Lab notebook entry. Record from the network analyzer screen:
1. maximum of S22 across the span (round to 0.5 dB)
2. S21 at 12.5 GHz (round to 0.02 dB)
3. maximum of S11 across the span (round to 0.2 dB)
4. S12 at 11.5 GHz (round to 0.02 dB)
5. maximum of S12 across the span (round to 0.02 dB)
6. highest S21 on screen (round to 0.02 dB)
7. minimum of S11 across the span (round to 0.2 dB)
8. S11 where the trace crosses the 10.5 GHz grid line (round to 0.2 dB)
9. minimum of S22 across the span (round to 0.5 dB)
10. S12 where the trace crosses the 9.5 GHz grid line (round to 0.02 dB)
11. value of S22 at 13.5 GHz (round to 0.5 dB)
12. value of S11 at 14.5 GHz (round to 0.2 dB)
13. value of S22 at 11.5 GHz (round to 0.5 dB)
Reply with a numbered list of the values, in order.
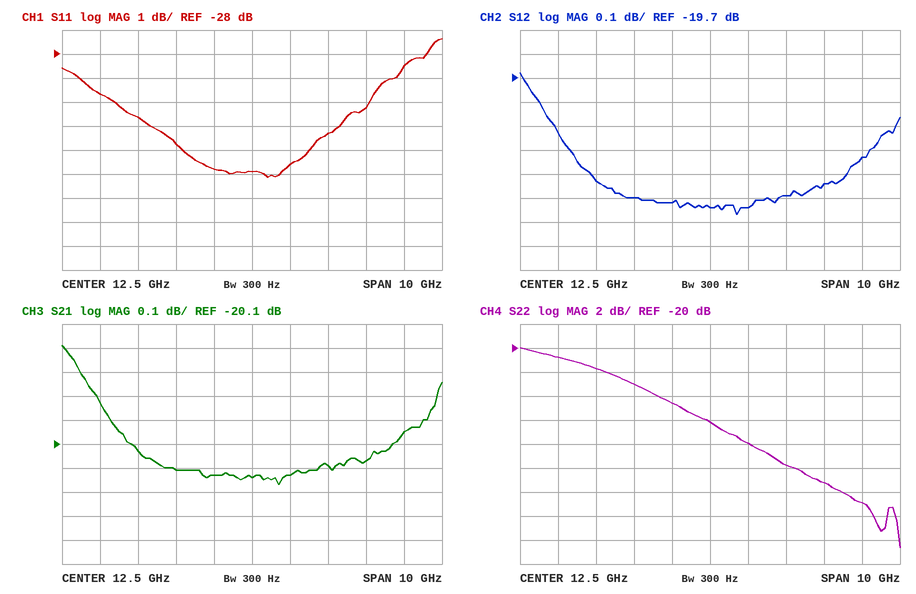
1. -20.0 dB
2. -20.24 dB
3. -27.4 dB
4. -20.22 dB
5. -19.68 dB
6. -19.68 dB
7. -33.2 dB
8. -31.8 dB
9. -36.5 dB
10. -20.12 dB
11. -28.0 dB
12. -31.4 dB
13. -24.5 dB
